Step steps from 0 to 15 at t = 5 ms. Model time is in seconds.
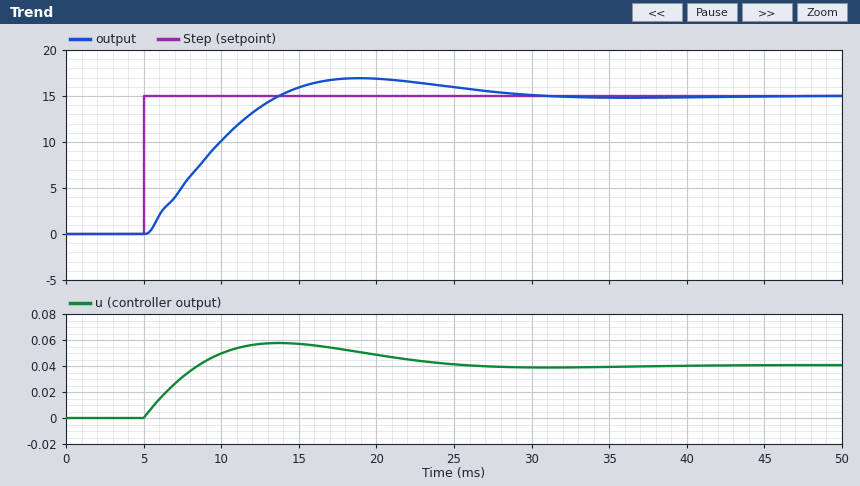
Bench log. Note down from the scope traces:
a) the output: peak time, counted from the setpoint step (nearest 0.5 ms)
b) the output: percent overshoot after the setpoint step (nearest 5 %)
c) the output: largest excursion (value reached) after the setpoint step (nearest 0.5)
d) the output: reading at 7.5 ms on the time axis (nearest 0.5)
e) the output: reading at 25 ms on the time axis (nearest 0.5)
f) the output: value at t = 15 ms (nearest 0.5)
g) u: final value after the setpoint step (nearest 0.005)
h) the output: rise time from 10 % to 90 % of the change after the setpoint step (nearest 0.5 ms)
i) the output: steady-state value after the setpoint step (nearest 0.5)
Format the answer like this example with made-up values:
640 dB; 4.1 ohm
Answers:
14.0 ms; 15 %; 17.0; 5.0; 16.0; 16.0; 0.040; 6.5 ms; 15.0
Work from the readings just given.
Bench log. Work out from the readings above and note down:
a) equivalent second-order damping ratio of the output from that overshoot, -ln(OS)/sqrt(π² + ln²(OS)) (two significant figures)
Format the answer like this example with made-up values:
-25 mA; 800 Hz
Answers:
0.52
